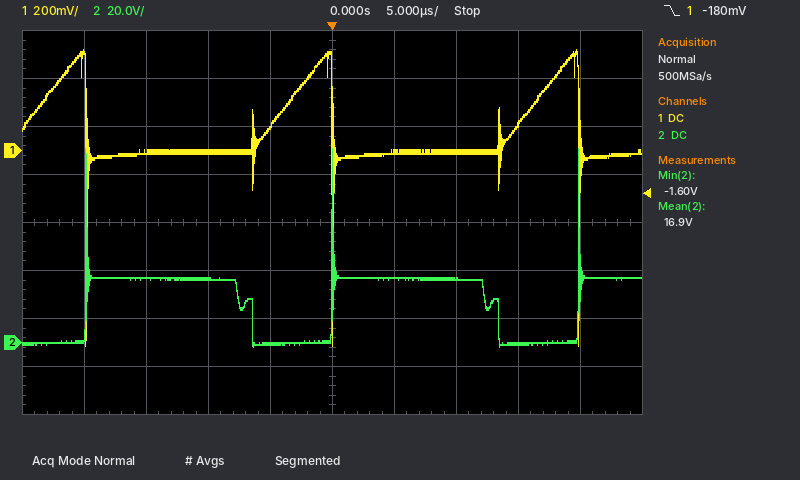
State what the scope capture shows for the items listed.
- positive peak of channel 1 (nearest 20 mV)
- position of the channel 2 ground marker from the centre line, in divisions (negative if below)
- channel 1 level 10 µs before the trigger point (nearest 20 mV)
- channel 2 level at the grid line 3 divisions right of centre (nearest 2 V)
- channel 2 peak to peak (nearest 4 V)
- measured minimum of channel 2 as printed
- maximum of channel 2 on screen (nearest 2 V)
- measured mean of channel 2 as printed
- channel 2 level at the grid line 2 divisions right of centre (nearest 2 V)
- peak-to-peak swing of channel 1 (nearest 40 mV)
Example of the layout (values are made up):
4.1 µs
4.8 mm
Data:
420 mV
-2.5 div
0 mV
0 V
84 V
-1.60 V
80 V
16.9 V
26 V
1.24 V
